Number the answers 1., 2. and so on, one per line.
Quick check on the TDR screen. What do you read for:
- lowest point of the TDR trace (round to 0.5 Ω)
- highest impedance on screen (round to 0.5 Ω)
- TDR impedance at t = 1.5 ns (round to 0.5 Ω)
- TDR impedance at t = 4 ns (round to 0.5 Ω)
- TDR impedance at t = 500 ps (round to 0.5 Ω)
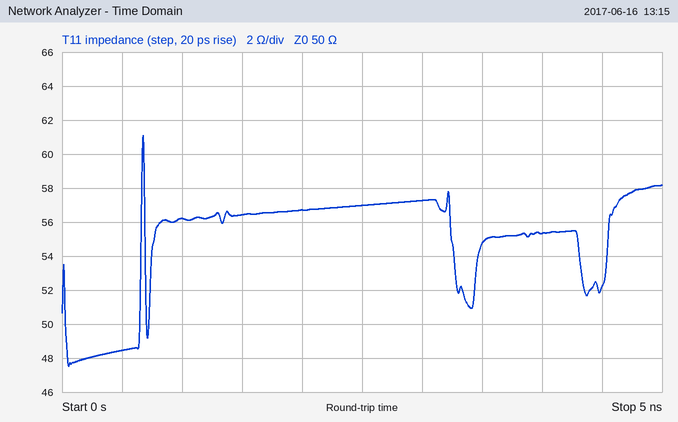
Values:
1. 47.5 Ω
2. 61.0 Ω
3. 56.5 Ω
4. 55.5 Ω
5. 48.5 Ω
